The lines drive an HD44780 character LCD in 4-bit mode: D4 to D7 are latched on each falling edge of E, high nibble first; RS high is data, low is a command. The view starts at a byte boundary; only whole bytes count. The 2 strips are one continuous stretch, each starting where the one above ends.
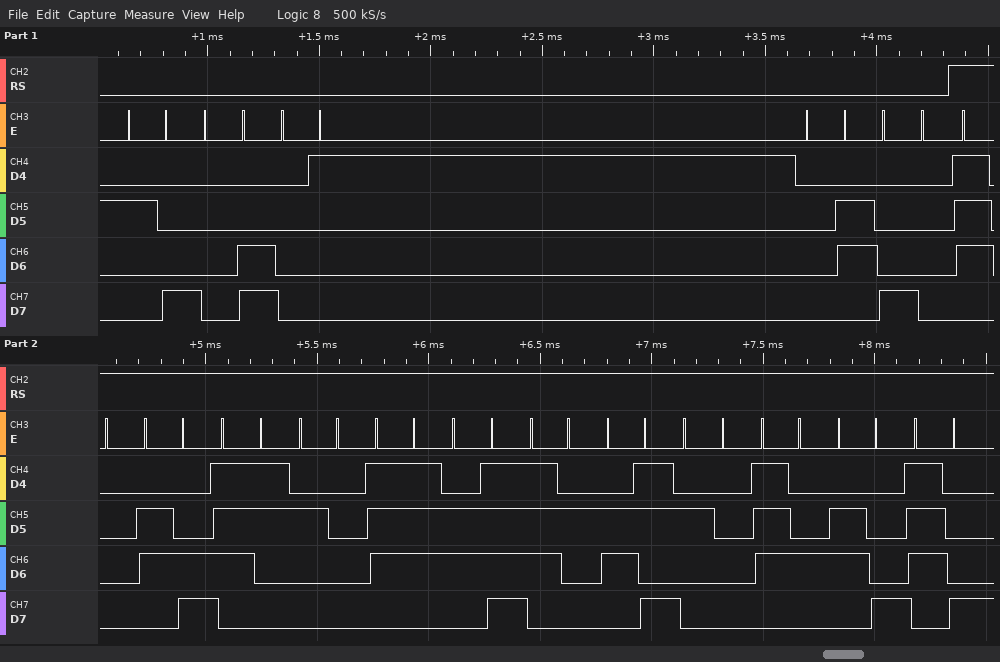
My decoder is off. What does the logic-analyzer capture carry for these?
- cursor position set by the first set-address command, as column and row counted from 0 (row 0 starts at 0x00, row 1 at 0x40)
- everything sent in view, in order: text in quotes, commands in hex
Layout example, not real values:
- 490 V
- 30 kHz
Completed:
- column 0, row 0
- 0x28 0x0C 0x01 0x06 0x80 "pls work thx"
